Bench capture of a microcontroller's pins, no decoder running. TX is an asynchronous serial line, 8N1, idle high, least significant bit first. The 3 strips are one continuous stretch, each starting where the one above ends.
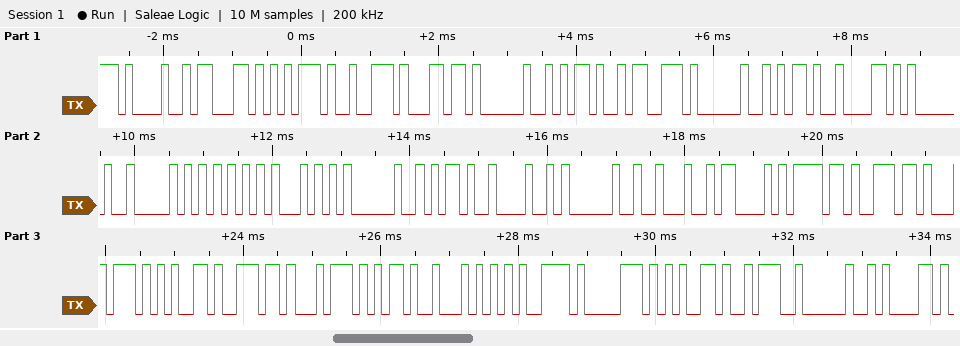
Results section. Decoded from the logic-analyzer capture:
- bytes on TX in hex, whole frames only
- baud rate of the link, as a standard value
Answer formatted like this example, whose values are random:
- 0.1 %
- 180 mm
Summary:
- 21 63 75 72 6C 20 2D 73 20 2D 58 20 50 55 54 20 2D 48 20 22 43 6F 6E 74 65 6E 74 2D 54 79 70 65 3A 20 61
- 9600 baud
